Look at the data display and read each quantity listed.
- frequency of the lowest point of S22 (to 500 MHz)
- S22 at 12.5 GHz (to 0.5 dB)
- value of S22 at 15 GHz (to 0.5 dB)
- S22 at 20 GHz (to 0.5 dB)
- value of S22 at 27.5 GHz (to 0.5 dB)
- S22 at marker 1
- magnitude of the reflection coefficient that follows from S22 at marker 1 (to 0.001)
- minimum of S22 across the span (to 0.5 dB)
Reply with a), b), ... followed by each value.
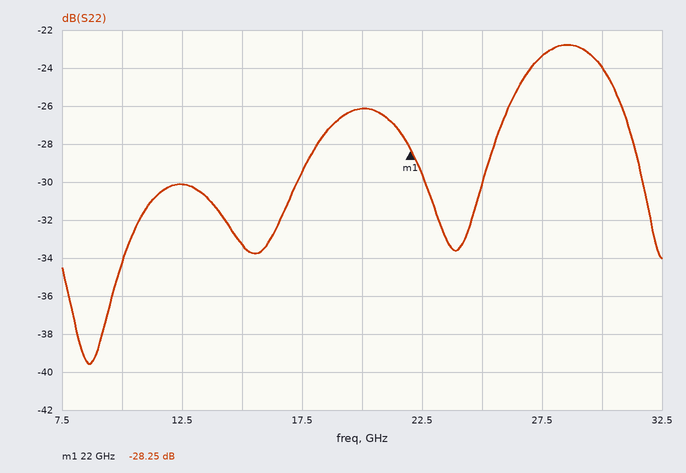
a) 8.5 GHz
b) -30.0 dB
c) -33.5 dB
d) -26.0 dB
e) -23.5 dB
f) -28.25 dB
g) 0.039
h) -39.5 dB
